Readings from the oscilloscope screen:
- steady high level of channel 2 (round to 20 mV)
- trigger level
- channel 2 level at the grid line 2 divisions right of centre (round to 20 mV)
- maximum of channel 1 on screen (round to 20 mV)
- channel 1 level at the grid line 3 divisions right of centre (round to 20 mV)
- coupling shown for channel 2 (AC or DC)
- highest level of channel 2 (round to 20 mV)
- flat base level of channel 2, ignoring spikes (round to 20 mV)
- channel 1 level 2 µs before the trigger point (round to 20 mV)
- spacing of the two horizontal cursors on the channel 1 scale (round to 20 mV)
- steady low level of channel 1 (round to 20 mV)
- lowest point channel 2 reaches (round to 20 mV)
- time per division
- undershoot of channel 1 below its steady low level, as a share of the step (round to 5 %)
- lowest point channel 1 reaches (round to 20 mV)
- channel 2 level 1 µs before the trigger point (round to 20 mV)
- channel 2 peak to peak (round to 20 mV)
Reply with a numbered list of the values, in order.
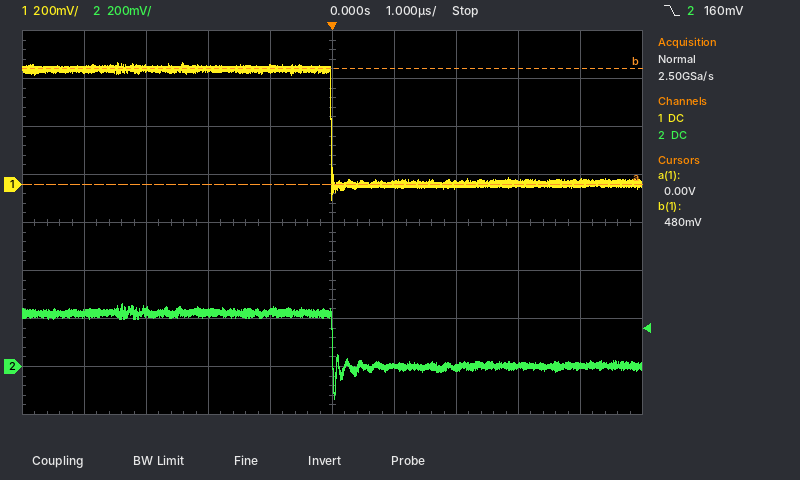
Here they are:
1. 220 mV
2. 160 mV
3. 0 mV
4. 500 mV
5. 0 mV
6. DC
7. 260 mV
8. 0 mV
9. 480 mV
10. 480 mV
11. 0 mV
12. -140 mV
13. 1 µs
14. 15 %
15. -60 mV
16. 220 mV
17. 400 mV
